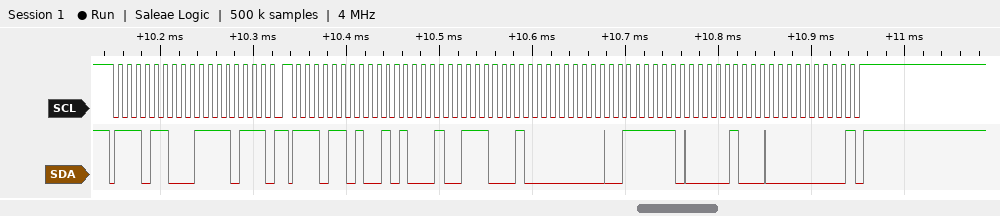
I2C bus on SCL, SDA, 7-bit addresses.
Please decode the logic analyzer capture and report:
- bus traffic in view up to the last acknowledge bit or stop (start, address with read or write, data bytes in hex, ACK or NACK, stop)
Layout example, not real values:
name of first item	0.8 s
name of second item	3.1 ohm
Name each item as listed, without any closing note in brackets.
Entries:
bus traffic in view up to the last acknowledge bit or stop	start, address 76 write ACK, F7 ACK, repeated start, address 76 read ACK, 51 ACK, 71 ACK, 00 ACK, 7E ACK, 08 ACK, 00 NACK, stop
